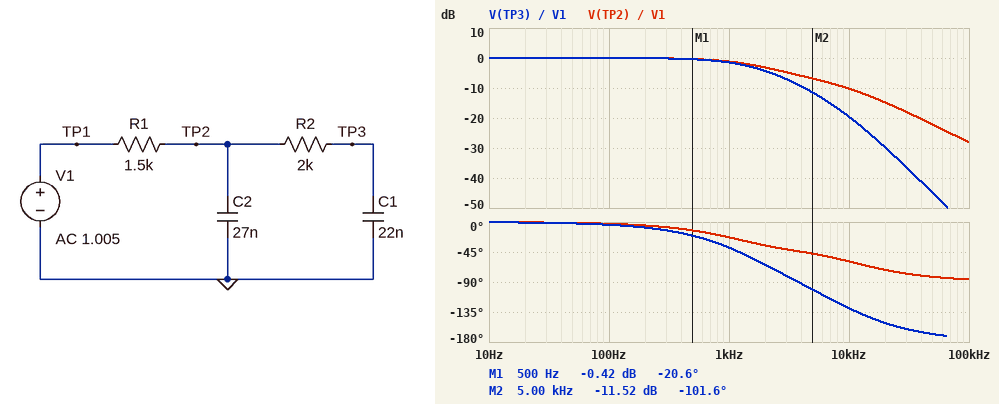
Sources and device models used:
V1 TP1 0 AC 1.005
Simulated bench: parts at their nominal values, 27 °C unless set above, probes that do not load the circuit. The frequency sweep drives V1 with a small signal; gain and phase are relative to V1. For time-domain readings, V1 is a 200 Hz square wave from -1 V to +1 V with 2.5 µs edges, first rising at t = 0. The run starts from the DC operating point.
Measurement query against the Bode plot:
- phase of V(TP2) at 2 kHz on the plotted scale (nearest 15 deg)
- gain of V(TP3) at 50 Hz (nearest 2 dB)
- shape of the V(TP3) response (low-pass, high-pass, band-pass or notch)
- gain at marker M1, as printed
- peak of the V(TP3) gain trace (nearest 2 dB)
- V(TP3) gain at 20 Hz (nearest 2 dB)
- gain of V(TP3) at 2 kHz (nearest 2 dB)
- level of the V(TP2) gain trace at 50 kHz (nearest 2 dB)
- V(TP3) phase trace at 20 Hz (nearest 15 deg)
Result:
-30 deg
0 dB
low-pass
-0.42 dB
0 dB
0 dB
-4 dB
-22 dB
0 deg
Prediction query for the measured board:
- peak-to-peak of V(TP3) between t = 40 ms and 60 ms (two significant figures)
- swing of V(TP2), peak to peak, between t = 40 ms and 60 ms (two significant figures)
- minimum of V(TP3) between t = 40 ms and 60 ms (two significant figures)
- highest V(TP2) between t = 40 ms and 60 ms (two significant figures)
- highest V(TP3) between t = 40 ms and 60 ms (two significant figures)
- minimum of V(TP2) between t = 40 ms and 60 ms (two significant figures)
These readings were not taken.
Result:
2.0 V
2.0 V
-1.0 V
1.0 V
1.0 V
-1.0 V
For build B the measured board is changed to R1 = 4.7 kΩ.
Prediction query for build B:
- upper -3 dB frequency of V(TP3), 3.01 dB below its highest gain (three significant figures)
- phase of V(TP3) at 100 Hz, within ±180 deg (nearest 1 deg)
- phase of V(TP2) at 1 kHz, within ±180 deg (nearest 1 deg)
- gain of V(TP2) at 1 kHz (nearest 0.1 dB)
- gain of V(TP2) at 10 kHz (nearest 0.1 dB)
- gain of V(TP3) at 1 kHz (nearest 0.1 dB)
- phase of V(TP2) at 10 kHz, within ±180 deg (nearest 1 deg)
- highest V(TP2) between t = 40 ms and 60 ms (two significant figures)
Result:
626 Hz
-10 deg
-50 deg
-5.2 dB
-19.3 dB
-5.5 dB
-71 deg
1.0 V
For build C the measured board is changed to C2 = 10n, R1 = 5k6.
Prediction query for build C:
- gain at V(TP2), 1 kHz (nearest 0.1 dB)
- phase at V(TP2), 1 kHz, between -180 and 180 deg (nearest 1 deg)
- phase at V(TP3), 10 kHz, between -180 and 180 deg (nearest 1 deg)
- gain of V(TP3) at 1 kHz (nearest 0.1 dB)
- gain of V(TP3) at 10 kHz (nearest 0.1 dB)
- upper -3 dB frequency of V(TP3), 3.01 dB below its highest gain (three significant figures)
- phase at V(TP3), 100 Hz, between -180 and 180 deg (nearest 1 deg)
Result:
-4.1 dB
-42 deg
-122 deg
-4.4 dB
-24.4 dB
750 Hz
-8 deg
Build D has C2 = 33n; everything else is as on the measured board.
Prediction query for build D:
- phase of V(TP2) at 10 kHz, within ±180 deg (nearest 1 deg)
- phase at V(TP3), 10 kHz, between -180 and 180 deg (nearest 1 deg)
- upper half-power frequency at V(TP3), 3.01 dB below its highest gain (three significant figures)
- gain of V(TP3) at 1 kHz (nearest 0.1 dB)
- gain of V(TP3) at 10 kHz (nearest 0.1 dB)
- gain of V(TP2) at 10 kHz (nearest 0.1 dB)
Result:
-64 deg
-134 deg
1.45 kHz
-1.7 dB
-20.8 dB
-11.5 dB
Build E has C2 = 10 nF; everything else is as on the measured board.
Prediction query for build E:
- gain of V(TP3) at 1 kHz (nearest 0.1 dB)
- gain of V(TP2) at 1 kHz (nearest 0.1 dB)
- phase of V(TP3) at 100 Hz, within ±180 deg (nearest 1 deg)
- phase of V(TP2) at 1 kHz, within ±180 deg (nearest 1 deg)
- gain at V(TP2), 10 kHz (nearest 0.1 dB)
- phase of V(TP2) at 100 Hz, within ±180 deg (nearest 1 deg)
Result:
-1.1 dB
-0.8 dB
-3 deg
-15 deg
-6.2 dB
-2 deg
